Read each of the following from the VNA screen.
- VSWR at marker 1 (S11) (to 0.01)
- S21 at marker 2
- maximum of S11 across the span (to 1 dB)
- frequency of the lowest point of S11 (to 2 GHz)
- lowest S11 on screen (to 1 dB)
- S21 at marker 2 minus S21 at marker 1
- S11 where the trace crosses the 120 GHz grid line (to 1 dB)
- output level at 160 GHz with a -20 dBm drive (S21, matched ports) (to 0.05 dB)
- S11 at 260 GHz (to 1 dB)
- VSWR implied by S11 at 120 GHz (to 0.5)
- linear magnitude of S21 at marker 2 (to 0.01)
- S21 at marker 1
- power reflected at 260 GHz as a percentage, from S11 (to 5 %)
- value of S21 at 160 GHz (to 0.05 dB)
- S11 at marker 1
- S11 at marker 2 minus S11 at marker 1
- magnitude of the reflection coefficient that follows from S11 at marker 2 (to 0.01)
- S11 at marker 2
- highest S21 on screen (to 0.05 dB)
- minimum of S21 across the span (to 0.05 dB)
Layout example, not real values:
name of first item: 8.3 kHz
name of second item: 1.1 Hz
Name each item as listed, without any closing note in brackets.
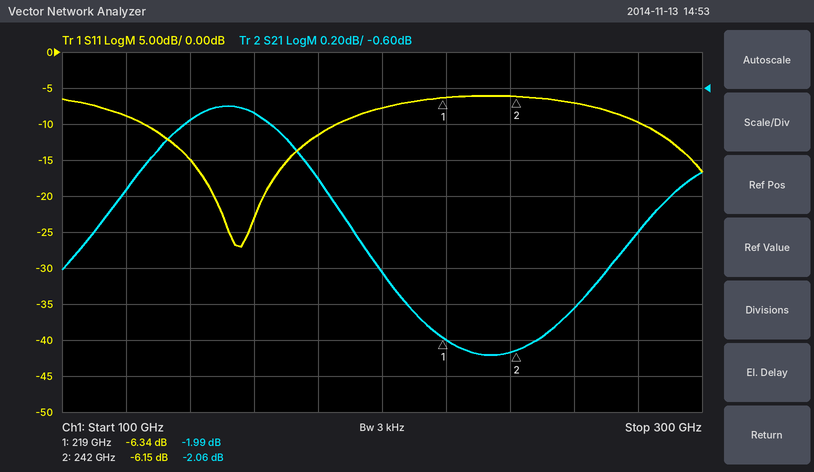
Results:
VSWR at marker 1 (S11): 2.86
S21 at marker 2: -2.06 dB
maximum of S11 across the span: -6 dB
frequency of the lowest point of S11: 156 GHz
lowest S11 on screen: -27 dB
S21 at marker 2 minus S21 at marker 1: -0.07 dB
S11 where the trace crosses the 120 GHz grid line: -9 dB
output level at 160 GHz with a -20 dBm drive (S21, matched ports): -20.75 dBm
S11 at 260 GHz: -7 dB
VSWR implied by S11 at 120 GHz: 2.0
linear magnitude of S21 at marker 2: 0.79
S21 at marker 1: -1.99 dB
power reflected at 260 GHz as a percentage, from S11: 20 %
value of S21 at 160 GHz: -0.75 dB
S11 at marker 1: -6.34 dB
S11 at marker 2 minus S11 at marker 1: 0.19 dB
magnitude of the reflection coefficient that follows from S11 at marker 2: 0.49
S11 at marker 2: -6.15 dB
highest S21 on screen: -0.70 dB
minimum of S21 across the span: -2.10 dB
